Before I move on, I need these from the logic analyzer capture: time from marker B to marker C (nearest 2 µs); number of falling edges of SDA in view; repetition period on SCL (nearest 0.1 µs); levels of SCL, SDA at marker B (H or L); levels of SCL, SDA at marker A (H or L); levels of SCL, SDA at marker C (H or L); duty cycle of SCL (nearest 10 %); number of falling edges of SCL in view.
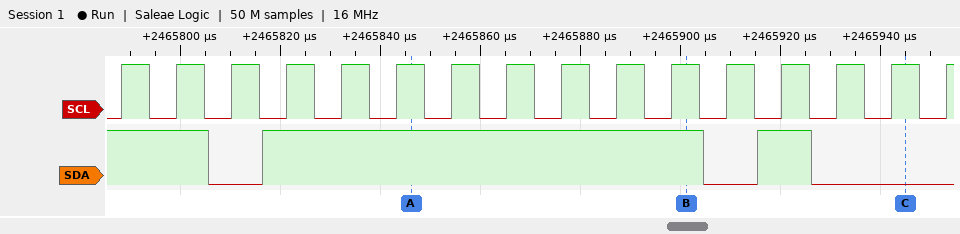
44 µs
3
11 µs
SCL=H, SDA=H
SCL=H, SDA=H
SCL=H, SDA=L
50 %
15
